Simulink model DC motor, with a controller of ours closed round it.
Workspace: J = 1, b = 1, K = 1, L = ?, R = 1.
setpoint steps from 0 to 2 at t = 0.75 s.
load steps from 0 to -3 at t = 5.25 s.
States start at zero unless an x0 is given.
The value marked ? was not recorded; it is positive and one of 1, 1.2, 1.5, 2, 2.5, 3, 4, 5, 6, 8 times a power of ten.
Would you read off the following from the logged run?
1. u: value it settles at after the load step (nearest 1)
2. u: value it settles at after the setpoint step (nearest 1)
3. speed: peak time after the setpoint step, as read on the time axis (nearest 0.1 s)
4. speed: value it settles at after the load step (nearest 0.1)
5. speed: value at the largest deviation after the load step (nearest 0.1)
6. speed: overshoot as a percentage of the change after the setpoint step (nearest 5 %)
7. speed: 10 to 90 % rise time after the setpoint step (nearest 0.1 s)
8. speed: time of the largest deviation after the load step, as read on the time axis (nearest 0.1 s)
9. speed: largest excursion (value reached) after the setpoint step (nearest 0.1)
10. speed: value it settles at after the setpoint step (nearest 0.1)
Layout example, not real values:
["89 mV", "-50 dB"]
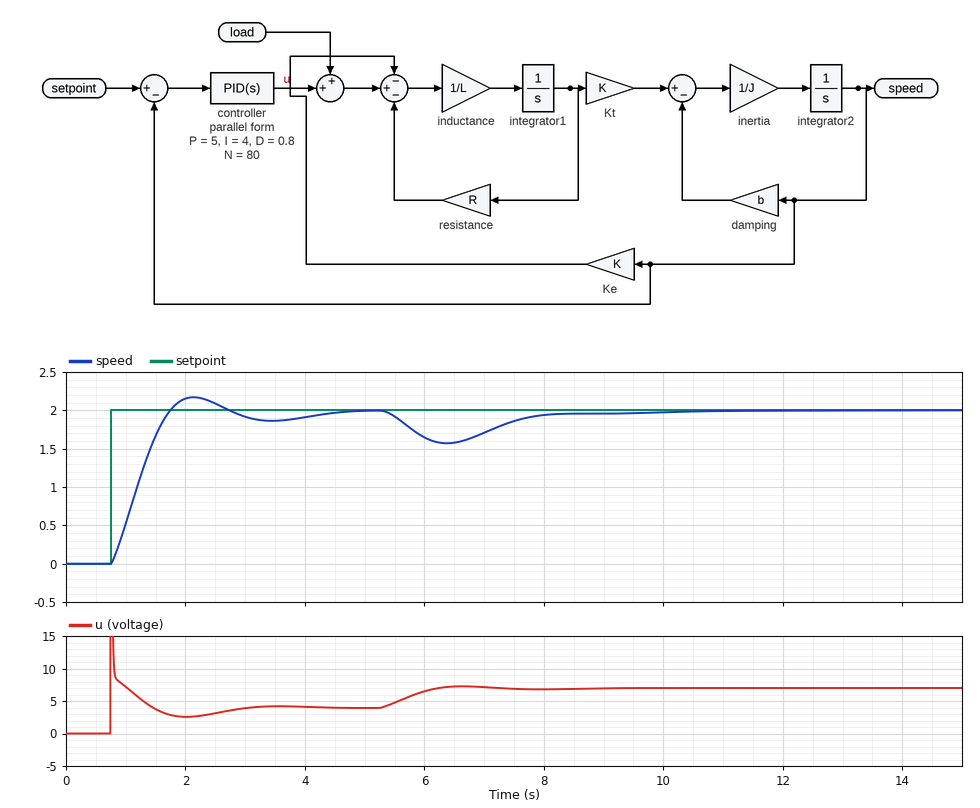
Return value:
["7", "4", "2.1 s", "2.0", "1.6", "10 %", "0.7 s", "6.4 s", "2.2", "2.0"]
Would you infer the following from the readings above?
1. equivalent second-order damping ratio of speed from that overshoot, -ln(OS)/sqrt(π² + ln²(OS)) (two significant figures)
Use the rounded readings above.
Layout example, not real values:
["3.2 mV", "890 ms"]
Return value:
["0.59"]
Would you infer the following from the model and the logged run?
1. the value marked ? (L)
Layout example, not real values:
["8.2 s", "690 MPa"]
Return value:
["1"]
